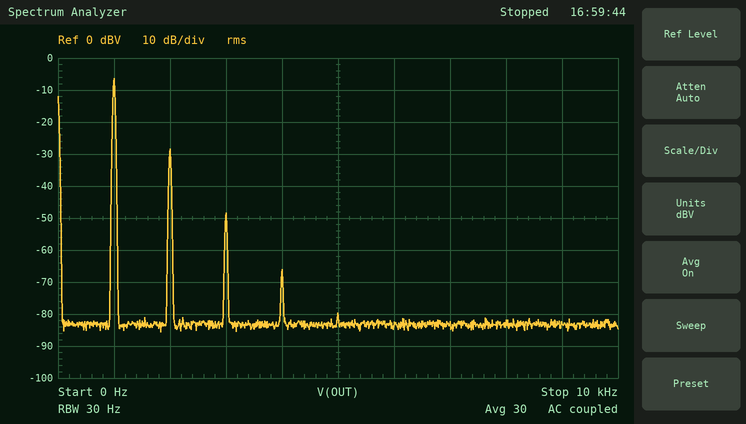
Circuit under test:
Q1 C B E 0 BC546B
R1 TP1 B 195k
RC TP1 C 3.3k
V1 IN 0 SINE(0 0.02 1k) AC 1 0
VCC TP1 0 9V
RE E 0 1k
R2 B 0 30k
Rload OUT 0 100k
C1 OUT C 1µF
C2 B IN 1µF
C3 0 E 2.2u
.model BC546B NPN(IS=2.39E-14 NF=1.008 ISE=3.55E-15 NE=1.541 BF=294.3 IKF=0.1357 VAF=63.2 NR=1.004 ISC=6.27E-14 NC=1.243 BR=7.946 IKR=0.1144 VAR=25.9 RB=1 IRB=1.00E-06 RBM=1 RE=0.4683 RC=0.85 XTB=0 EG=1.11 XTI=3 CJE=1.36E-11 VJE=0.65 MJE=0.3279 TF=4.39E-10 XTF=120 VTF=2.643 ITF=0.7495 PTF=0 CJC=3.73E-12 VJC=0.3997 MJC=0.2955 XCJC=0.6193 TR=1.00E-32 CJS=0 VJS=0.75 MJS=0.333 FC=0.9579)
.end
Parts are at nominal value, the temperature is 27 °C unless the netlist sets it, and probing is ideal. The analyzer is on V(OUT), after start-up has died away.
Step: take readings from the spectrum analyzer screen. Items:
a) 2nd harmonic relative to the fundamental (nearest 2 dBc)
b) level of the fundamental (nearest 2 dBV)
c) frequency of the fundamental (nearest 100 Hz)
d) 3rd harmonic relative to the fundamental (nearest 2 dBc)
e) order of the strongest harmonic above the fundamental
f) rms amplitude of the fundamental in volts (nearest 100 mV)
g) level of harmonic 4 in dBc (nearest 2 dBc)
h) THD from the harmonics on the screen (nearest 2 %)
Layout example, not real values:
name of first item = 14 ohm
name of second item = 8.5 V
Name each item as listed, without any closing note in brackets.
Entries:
2nd harmonic relative to the fundamental = -22 dBc
level of the fundamental = -6 dBV
frequency of the fundamental = 1.0 kHz
3rd harmonic relative to the fundamental = -42 dBc
order of the strongest harmonic above the fundamental = 2
rms amplitude of the fundamental in volts = 500 mV
level of harmonic 4 in dBc = -60 dBc
THD from the harmonics on the screen = 8 %
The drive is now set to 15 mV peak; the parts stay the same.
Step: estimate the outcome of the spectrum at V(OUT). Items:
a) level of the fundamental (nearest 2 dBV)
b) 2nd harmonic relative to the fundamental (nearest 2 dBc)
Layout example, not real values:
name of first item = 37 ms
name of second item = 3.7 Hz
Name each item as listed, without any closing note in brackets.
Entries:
level of the fundamental = -8 dBV
2nd harmonic relative to the fundamental = -24 dBc
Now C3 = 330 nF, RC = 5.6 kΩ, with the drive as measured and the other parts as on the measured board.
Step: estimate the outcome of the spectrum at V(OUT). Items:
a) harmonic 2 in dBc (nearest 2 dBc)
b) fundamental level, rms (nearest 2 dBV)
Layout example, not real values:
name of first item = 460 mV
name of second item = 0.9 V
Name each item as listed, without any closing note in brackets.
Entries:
harmonic 2 in dBc = -48 dBc
fundamental level, rms = -16 dBV
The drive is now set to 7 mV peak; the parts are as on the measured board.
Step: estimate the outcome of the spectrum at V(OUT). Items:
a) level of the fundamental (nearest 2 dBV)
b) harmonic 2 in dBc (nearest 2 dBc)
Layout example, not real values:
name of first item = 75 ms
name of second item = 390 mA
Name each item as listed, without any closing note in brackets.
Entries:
level of the fundamental = -16 dBV
harmonic 2 in dBc = -32 dBc
